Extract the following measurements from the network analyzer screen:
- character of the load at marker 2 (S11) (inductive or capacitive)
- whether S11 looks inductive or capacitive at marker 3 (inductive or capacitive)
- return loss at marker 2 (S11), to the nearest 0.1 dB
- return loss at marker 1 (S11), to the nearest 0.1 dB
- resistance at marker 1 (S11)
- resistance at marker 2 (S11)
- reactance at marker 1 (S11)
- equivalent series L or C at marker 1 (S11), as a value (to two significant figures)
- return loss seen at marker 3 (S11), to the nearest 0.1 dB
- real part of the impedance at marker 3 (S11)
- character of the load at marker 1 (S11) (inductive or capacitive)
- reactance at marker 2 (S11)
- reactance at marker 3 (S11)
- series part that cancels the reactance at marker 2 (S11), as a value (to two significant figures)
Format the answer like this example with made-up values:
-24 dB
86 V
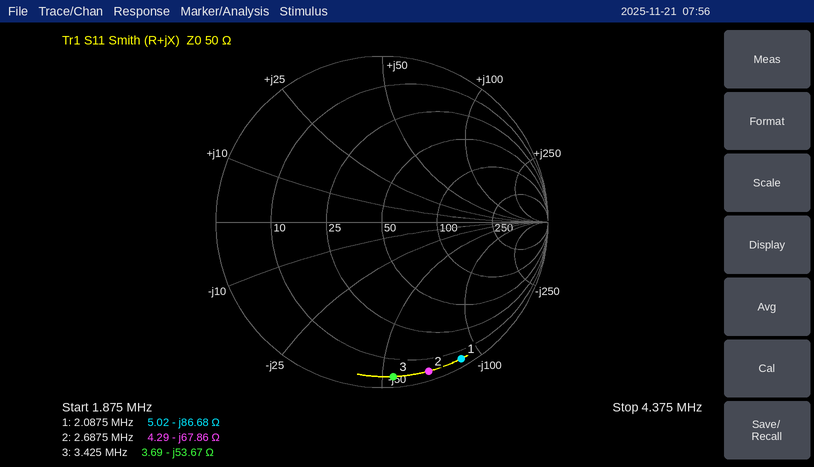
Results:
capacitive
capacitive
0.5 dB
0.4 dB
5.02 Ω
4.29 Ω
-86.68 Ω
880 pF
0.6 dB
3.69 Ω
capacitive
-67.86 Ω
-53.67 Ω
4.0 µH
